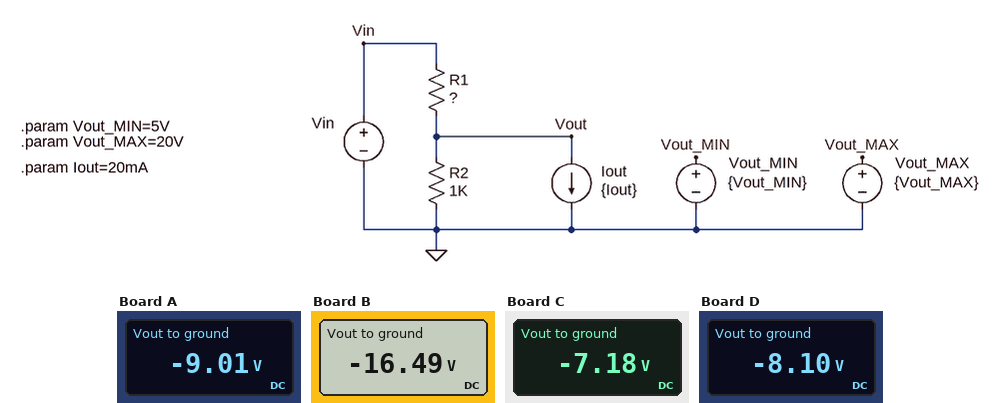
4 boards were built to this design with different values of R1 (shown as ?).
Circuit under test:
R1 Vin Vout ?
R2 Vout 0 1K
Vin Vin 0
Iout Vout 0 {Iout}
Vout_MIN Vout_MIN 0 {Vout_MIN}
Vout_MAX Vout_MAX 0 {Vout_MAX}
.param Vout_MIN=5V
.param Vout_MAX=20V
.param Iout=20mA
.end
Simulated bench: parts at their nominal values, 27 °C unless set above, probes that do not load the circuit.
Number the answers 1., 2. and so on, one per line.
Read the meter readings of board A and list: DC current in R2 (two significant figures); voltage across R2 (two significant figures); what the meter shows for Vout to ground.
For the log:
1. 9.0 mA
2. 9.0 V
3. -9.01 V
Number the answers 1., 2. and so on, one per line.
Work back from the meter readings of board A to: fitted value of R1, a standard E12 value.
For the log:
1. 820 Ω
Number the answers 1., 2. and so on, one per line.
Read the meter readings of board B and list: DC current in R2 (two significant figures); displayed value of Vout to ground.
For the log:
1. 16 mA
2. -16.49 V
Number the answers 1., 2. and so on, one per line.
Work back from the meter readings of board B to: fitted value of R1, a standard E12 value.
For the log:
1. 4.7 kΩ
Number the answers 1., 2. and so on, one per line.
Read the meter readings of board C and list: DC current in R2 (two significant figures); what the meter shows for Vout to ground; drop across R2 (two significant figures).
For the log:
1. 7.2 mA
2. -7.18 V
3. 7.2 V
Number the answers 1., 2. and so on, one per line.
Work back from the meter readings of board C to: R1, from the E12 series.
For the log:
1. 560 Ω
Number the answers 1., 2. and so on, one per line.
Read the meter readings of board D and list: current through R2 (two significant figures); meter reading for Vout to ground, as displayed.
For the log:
1. 8.1 mA
2. -8.10 V
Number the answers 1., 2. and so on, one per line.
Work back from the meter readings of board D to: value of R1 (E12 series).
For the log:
1. 680 Ω
